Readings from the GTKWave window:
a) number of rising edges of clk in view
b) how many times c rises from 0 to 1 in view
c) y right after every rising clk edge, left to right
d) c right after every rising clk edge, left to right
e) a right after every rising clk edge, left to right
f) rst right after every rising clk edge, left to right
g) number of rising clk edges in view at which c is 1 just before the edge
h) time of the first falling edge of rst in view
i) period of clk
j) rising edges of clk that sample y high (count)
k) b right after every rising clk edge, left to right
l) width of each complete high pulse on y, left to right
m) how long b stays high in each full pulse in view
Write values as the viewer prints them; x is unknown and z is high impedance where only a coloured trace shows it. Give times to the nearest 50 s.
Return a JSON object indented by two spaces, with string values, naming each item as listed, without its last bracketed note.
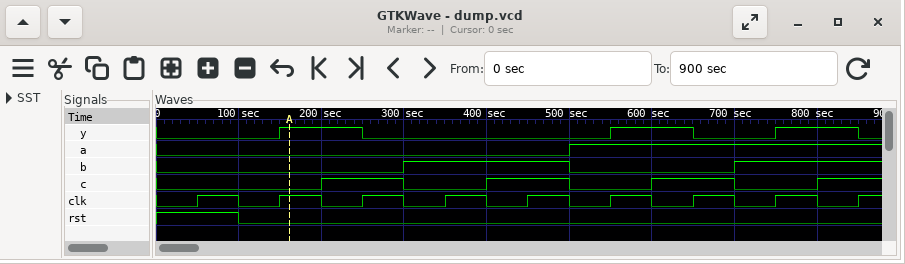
{
  "number of rising edges of clk in view": "9",
  "how many times c rises from 0 to 1 in view": "4",
  "y right after every rising clk edge, left to right": "0 1 0 0 0 1 0 1 0",
  "c right after every rising clk edge, left to right": "0 0 1 0 1 0 1 0 1",
  "a right after every rising clk edge, left to right": "0 0 0 0 0 1 1 1 1",
  "rst right after every rising clk edge, left to right": "1 0 0 0 0 0 0 0 0",
  "number of rising clk edges in view at which c is 1 just before the edge": "4",
  "time of the first falling edge of rst in view": "100 s",
  "period of clk": "100 s",
  "rising edges of clk that sample y high": "3",
  "b right after every rising clk edge, left to right": "0 0 0 1 1 0 0 1 1",
  "width of each complete high pulse on y, left to right": "100 s, 100 s, 100 s",
  "how long b stays high in each full pulse in view": "200 s"
}
